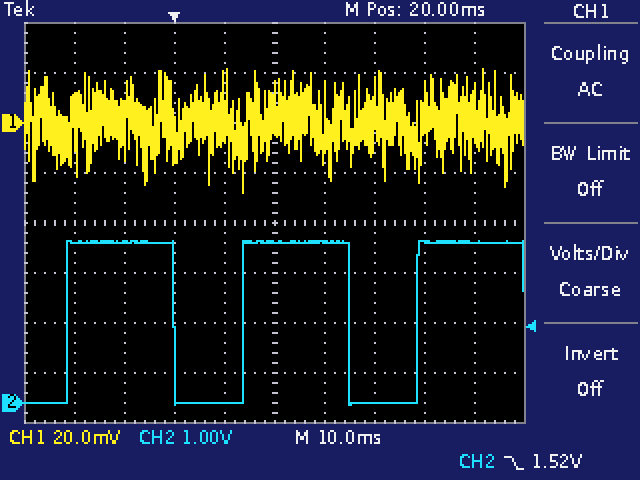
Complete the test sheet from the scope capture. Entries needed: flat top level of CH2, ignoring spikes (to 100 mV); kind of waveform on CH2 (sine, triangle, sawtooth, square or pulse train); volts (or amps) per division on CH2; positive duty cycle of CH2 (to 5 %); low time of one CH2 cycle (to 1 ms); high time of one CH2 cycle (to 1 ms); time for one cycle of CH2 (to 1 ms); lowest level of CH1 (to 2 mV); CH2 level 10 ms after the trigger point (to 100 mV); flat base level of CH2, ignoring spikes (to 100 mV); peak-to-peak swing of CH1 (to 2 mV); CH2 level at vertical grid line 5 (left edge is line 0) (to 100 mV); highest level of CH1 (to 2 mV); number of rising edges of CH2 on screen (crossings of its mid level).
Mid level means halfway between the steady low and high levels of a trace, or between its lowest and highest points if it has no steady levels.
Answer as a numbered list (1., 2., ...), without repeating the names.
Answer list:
1. 3.2 V
2. pulse train
3. 1 V
4. 60 %
5. 14 ms
6. 21 ms
7. 35 ms
8. -28 mV
9. 0.0 V
10. 0.0 V
11. 50 mV
12. 3.2 V
13. 22 mV
14. 3
